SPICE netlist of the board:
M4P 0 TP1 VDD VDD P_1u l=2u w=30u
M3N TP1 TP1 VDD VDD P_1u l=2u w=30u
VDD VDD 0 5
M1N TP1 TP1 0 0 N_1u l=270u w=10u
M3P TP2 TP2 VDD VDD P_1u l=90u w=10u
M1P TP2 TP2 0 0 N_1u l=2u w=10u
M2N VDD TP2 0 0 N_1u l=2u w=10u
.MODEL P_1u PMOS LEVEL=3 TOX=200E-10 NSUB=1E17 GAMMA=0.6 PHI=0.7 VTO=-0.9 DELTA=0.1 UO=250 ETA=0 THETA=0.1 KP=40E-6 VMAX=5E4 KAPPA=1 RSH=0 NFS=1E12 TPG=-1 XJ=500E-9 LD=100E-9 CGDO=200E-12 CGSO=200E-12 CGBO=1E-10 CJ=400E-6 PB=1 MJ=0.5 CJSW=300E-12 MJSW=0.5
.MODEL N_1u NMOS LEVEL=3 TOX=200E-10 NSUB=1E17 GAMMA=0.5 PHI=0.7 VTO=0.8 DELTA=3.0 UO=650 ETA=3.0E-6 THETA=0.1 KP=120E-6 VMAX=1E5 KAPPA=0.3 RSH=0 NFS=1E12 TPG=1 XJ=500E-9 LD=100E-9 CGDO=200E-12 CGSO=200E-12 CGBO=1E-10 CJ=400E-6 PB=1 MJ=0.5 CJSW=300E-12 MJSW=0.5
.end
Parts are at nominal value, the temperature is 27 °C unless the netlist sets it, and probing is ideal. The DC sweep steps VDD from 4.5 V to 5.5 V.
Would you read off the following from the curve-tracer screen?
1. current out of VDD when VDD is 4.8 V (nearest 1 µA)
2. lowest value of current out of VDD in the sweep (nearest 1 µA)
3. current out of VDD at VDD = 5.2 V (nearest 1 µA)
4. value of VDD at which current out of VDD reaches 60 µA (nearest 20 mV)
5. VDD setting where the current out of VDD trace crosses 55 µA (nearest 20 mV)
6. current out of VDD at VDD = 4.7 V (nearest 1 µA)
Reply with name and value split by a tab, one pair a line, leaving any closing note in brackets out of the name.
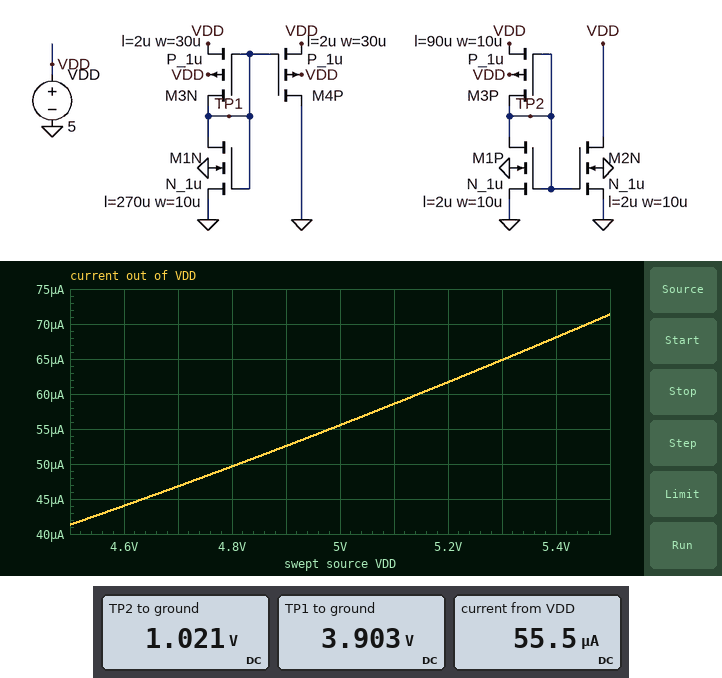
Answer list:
current out of VDD when VDD is 4.8 V	50 µA
lowest value of current out of VDD in the sweep	41 µA
current out of VDD at VDD = 5.2 V	62 µA
value of VDD at which current out of VDD reaches 60 µA	5.14 V
VDD setting where the current out of VDD trace crosses 55 µA	4.98 V
current out of VDD at VDD = 4.7 V	47 µA
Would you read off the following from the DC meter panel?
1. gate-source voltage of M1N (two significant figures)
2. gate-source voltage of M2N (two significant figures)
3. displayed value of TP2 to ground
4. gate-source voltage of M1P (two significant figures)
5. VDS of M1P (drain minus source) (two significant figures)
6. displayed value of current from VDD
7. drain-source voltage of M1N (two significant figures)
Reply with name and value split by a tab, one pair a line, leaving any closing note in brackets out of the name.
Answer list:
gate-source voltage of M1N	3.9 V
gate-source voltage of M2N	1.0 V
displayed value of TP2 to ground	1.021 V
gate-source voltage of M1P	1.0 V
VDS of M1P (drain minus source)	1.0 V
displayed value of current from VDD	55.5 µA
drain-source voltage of M1N	3.9 V
